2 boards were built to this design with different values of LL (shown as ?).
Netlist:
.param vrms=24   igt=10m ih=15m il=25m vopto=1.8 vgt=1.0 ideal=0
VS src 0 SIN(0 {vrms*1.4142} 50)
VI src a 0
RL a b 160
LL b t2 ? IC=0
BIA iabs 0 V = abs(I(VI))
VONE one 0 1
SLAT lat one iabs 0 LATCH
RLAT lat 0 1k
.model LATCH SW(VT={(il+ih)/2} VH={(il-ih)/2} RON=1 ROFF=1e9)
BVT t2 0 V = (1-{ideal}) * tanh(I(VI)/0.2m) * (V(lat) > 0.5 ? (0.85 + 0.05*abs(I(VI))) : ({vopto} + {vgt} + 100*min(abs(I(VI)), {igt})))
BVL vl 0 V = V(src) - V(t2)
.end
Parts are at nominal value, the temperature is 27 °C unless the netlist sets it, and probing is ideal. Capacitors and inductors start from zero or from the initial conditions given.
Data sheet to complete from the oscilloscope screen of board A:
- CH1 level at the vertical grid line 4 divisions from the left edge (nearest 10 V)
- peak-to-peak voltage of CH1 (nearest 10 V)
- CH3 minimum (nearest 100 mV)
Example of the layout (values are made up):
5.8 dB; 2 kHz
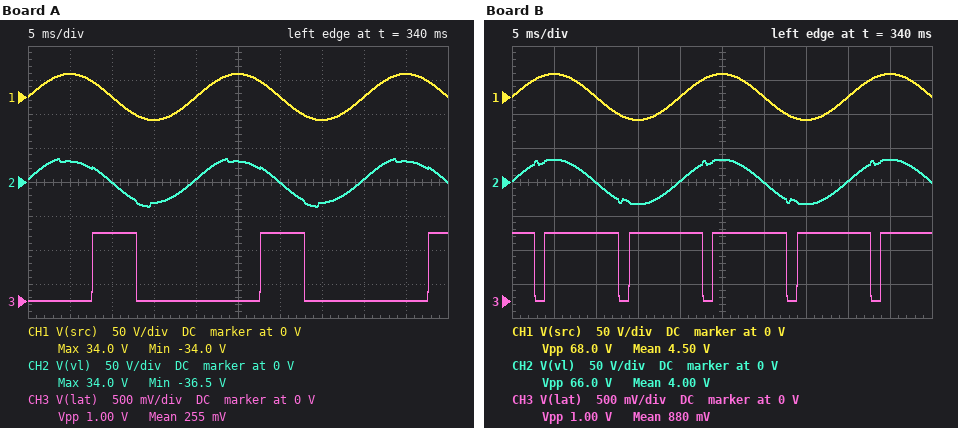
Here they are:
0 V; 70 V; 0 V
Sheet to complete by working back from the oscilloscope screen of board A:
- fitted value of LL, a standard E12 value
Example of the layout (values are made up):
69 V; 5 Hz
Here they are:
3.9 H
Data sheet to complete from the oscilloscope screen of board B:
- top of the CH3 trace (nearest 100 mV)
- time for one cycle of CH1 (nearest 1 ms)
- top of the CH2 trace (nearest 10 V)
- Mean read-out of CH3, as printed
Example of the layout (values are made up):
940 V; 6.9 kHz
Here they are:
1.0 V; 20 ms; 30 V; 880 mV
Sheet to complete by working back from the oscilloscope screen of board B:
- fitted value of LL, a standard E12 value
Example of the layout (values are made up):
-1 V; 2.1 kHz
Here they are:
820 mH
